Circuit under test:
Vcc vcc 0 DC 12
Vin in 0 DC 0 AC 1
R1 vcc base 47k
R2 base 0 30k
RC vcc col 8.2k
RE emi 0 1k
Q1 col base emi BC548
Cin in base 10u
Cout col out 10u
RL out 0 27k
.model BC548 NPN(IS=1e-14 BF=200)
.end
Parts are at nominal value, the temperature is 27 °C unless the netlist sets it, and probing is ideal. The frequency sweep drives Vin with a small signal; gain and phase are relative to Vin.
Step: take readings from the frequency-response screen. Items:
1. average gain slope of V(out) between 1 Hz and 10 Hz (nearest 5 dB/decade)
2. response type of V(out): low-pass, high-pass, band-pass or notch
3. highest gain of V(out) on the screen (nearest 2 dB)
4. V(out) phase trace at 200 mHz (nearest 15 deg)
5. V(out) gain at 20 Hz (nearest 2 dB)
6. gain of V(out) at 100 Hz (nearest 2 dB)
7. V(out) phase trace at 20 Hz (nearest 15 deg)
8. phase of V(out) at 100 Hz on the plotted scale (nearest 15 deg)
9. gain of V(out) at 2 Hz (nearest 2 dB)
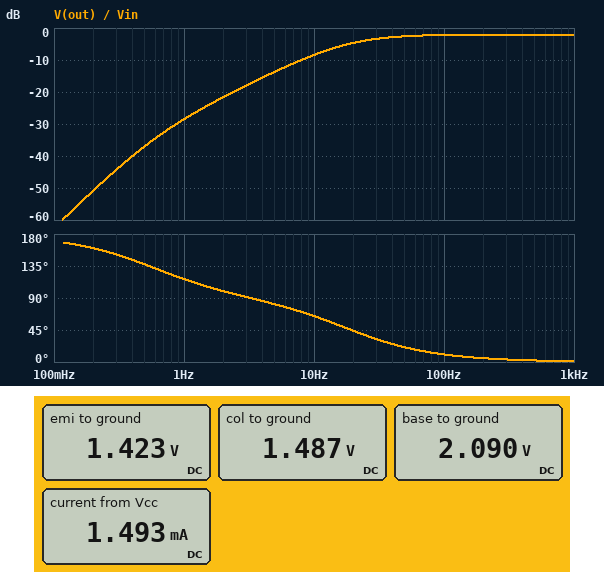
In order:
20 dB/decade
high-pass
-2 dB
165 deg
-4 dB
-2 dB
45 deg
15 deg
-22 dB
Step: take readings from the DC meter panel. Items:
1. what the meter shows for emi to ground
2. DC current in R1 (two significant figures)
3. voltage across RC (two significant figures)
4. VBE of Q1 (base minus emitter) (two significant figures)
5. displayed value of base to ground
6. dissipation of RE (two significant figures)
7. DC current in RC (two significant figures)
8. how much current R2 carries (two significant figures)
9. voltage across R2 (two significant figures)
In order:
1.423 V
210 µA
11 V
670 mV
2.090 V
2.0 mW
1.3 mA
70 µA
2.1 V
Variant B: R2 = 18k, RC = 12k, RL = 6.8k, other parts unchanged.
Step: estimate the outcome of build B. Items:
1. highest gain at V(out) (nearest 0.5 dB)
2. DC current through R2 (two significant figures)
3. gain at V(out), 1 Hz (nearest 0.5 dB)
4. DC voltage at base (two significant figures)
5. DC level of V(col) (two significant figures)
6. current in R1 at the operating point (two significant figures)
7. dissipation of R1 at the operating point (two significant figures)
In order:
-2.5 dB
94 µA
-35.5 dB
1.7 V
1.1 V
220 µA
2.3 mW
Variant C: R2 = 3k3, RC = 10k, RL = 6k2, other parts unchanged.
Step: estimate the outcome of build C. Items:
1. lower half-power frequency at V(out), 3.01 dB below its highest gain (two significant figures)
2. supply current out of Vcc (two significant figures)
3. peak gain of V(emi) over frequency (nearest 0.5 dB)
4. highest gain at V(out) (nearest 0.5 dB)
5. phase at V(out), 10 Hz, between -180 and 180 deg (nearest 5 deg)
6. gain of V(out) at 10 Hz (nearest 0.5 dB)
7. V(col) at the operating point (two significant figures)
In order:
5.4 Hz
410 µA
-1.0 dB
10.5 dB
-145 deg
9.5 dB
10 V
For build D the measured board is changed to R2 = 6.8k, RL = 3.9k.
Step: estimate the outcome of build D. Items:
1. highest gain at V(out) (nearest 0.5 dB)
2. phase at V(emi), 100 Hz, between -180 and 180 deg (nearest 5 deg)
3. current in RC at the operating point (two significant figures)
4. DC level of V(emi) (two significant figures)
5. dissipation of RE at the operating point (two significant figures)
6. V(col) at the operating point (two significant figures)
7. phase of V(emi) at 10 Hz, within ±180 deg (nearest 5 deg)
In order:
8.0 dB
0 deg
840 µA
840 mV
710 µW
5.1 V
15 deg
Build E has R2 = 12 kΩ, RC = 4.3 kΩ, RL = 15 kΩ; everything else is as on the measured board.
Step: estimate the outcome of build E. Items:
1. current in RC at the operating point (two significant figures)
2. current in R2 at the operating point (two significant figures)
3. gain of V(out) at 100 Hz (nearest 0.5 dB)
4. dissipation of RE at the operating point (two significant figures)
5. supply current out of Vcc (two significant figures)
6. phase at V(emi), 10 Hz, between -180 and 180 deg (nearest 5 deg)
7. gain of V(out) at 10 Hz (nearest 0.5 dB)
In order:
1.7 mA
200 µA
10.5 dB
2.9 mW
1.9 mA
10 deg
10.0 dB
